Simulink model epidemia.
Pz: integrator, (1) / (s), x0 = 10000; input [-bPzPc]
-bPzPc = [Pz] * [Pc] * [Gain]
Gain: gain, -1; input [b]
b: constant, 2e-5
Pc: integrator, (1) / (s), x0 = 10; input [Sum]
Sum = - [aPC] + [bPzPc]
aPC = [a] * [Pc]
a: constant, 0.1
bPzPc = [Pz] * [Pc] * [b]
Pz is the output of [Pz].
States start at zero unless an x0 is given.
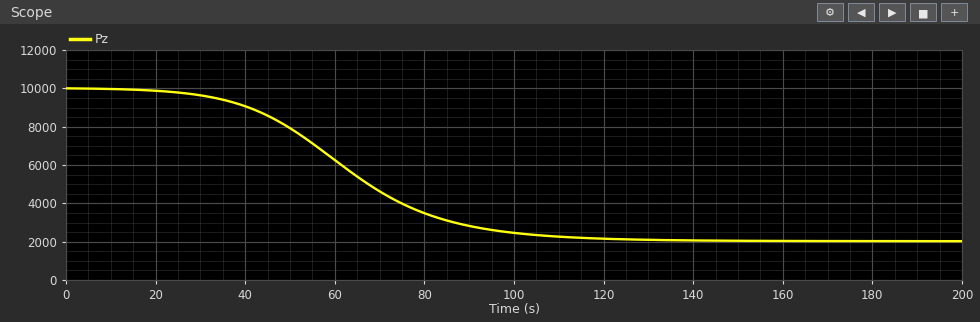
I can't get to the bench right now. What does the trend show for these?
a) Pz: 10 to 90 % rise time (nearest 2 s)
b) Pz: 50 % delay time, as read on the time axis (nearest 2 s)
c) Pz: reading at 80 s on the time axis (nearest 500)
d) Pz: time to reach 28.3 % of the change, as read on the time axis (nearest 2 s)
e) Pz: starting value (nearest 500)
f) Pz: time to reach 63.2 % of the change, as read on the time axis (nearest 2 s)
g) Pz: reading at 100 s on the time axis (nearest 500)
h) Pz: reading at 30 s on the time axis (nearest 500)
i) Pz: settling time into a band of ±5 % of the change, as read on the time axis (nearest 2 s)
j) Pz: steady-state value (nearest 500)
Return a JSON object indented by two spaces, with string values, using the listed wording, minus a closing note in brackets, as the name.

{
  "Pz: 10 to 90 % rise time": "52 s",
  "Pz: 50 % delay time, as read on the time axis": "62 s",
  "Pz: reading at 80 s on the time axis": "3500",
  "Pz: time to reach 28.3 % of the change, as read on the time axis": "52 s",
  "Pz: starting value": "10000",
  "Pz: time to reach 63.2 % of the change, as read on the time axis": "68 s",
  "Pz: reading at 100 s on the time axis": "2500",
  "Pz: reading at 30 s on the time axis": "9500",
  "Pz: settling time into a band of ±5 % of the change, as read on the time axis": "102 s",
  "Pz: steady-state value": "2000"
}
